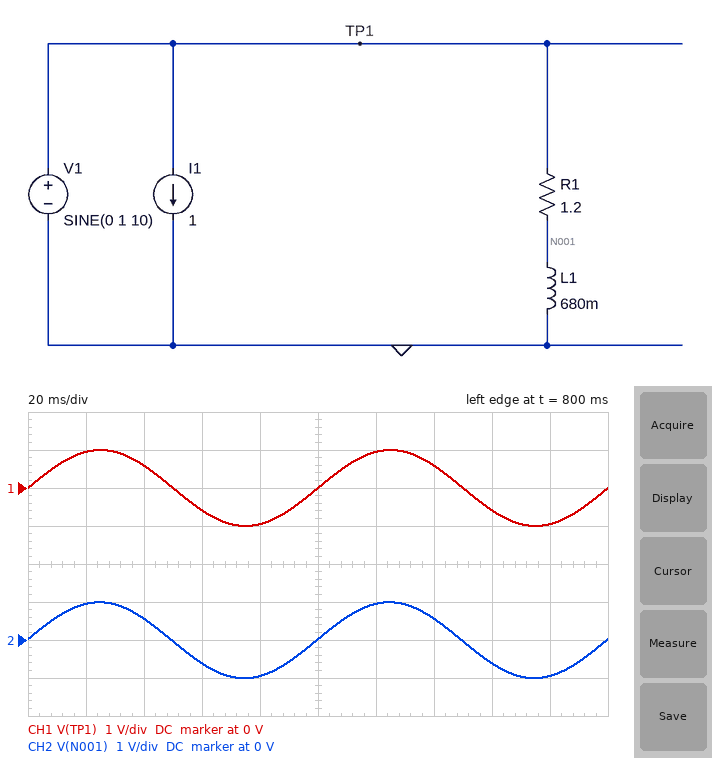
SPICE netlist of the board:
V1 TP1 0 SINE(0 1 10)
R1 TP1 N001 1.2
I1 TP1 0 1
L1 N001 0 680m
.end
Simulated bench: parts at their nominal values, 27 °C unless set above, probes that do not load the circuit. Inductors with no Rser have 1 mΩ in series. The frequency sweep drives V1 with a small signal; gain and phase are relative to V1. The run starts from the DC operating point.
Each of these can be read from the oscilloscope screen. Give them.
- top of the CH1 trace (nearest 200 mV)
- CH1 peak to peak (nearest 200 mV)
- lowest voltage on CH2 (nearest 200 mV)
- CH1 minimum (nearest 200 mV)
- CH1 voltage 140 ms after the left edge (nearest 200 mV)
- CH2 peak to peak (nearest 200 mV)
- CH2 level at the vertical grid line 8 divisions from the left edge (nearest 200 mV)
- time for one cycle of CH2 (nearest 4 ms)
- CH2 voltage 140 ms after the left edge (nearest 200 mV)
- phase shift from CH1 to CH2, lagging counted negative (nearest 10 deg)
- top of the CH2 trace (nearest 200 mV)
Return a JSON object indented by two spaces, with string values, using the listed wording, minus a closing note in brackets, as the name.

{
  "top of the CH1 trace": "1.0 V",
  "CH1 peak to peak": "2.0 V",
  "lowest voltage on CH2": "-1.0 V",
  "CH1 minimum": "-1.0 V",
  "CH1 voltage 140 ms after the left edge": "600 mV",
  "CH2 peak to peak": "2.0 V",
  "CH2 level at the vertical grid line 8 divisions from the left edge": "-600 mV",
  "time for one cycle of CH2": "100 ms",
  "CH2 voltage 140 ms after the left edge": "600 mV",
  "phase shift from CH1 to CH2, lagging counted negative": "0 deg",
  "top of the CH2 trace": "1.0 V"
}
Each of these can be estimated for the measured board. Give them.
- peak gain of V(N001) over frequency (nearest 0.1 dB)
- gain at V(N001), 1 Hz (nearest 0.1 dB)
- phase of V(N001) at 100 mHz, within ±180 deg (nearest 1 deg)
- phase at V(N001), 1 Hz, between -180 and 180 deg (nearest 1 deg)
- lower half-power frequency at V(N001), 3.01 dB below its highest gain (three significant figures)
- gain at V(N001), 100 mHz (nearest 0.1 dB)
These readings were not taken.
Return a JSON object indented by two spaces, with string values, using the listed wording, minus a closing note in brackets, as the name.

{
  "peak gain of V(N001) over frequency": "0 dB",
  "gain at V(N001), 1 Hz": "-0.3 dB",
  "phase of V(N001) at 100 mHz, within ±180 deg": "70 deg",
  "phase at V(N001), 1 Hz, between -180 and 180 deg": "16 deg",
  "lower half-power frequency at V(N001), 3.01 dB below its highest gain": "281 mHz",
  "gain at V(N001), 100 mHz": "-9.5 dB"
}
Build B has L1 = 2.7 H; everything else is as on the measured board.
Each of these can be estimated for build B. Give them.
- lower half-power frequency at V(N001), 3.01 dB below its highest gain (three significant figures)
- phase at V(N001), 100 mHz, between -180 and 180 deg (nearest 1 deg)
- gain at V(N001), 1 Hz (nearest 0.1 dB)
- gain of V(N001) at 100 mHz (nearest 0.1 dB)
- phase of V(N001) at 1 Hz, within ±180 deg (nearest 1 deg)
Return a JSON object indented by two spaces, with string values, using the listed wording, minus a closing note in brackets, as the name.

{
  "lower half-power frequency at V(N001), 3.01 dB below its highest gain": "70.8 mHz",
  "phase at V(N001), 100 mHz, between -180 and 180 deg": "35 deg",
  "gain at V(N001), 1 Hz": "0 dB",
  "gain of V(N001) at 100 mHz": "-1.8 dB",
  "phase of V(N001) at 1 Hz, within ±180 deg": "4 deg"
}
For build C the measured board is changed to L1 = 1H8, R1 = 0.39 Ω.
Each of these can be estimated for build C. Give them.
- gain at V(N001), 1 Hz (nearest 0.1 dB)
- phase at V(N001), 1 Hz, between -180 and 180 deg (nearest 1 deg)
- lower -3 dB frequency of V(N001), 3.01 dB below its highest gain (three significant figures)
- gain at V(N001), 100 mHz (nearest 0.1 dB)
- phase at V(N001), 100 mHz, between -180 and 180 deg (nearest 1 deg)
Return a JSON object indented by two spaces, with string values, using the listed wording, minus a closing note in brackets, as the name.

{
  "gain at V(N001), 1 Hz": "0 dB",
  "phase at V(N001), 1 Hz, between -180 and 180 deg": "2 deg",
  "lower -3 dB frequency of V(N001), 3.01 dB below its highest gain": "34.6 mHz",
  "gain at V(N001), 100 mHz": "-0.5 dB",
  "phase at V(N001), 100 mHz, between -180 and 180 deg": "19 deg"
}
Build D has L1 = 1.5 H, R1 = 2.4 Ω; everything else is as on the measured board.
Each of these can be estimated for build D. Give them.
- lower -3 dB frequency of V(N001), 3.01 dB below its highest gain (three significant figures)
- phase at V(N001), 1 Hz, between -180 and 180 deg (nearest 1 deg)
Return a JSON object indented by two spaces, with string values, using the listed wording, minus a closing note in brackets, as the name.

{
  "lower -3 dB frequency of V(N001), 3.01 dB below its highest gain": "255 mHz",
  "phase at V(N001), 1 Hz, between -180 and 180 deg": "14 deg"
}
